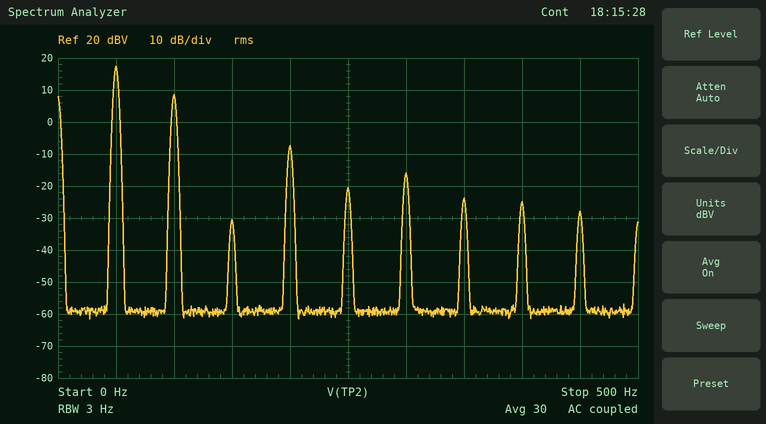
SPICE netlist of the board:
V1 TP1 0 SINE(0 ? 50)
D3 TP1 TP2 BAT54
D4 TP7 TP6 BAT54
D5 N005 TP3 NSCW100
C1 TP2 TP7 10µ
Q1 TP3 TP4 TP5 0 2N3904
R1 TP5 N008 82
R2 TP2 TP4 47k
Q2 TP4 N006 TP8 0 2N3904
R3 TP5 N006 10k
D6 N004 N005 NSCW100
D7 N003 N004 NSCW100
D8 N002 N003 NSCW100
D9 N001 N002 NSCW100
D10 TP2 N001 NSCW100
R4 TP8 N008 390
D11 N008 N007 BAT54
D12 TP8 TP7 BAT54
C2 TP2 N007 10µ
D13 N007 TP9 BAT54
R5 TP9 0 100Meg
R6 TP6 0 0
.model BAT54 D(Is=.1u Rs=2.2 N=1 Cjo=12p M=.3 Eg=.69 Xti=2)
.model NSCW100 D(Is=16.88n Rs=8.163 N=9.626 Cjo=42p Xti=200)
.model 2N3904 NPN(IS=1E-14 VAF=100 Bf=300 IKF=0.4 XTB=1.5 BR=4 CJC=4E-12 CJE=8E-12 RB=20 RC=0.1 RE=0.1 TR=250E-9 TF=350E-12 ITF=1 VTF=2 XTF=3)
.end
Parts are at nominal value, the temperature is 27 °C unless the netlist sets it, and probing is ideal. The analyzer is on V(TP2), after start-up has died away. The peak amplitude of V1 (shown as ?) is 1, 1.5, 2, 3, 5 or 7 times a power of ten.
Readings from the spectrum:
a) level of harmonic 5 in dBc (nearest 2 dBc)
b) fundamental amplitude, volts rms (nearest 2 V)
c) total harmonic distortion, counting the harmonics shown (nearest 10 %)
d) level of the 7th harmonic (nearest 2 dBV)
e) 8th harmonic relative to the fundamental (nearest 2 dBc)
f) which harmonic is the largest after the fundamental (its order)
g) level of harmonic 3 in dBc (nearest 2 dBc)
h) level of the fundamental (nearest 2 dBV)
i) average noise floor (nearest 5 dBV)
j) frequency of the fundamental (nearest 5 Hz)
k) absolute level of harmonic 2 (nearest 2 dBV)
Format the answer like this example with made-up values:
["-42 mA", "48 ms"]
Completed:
["-38 dBc", "8 V", "40 %", "-24 dBV", "-42 dBc", "2", "-48 dBc", "18 dBV", "-60 dBV", "50 Hz", "8 dBV"]
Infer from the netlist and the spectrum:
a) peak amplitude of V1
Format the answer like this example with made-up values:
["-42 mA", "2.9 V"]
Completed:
["20 V"]
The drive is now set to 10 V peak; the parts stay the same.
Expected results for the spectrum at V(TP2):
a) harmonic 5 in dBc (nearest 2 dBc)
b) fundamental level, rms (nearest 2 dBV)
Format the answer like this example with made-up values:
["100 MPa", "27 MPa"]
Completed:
["-34 dBc", "12 dBV"]
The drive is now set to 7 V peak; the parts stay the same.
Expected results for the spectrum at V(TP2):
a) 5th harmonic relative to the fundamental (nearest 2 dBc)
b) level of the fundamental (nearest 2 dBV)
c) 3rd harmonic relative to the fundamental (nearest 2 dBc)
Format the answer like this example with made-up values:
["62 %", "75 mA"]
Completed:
["-32 dBc", "8 dBV", "-40 dBc"]
